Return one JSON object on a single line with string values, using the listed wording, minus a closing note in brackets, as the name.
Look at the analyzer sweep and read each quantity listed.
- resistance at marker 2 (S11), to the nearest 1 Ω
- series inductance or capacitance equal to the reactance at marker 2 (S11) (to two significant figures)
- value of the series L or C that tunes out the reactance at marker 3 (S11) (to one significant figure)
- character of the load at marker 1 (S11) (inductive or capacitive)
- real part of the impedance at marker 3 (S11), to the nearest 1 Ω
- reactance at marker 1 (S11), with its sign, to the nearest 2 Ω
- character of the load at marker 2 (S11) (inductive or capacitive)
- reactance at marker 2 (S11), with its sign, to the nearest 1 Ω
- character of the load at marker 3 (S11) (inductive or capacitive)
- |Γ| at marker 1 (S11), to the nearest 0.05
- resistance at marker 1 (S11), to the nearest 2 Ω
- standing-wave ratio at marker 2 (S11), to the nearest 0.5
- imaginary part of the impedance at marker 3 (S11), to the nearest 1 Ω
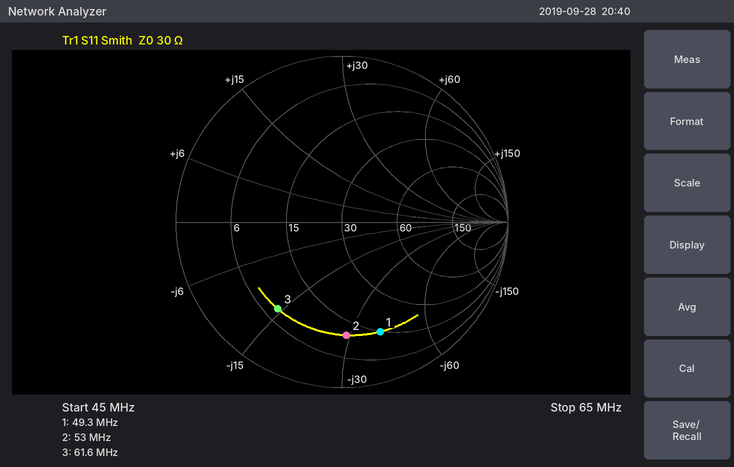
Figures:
{"resistance at marker 2 (S11), to the nearest 1 Ω": "11 Ω", "series inductance or capacitance equal to the reactance at marker 2 (S11)": "100 pF", "value of the series L or C that tunes out the reactance at marker 3 (S11)": "40 nH", "character of the load at marker 1 (S11)": "capacitive", "real part of the impedance at marker 3 (S11), to the nearest 1 Ω": "8 Ω", "reactance at marker 1 (S11), with its sign, to the nearest 2 Ω": "-38 Ω", "character of the load at marker 2 (S11)": "capacitive", "reactance at marker 2 (S11), with its sign, to the nearest 1 Ω": "-29 Ω", "character of the load at marker 3 (S11)": "capacitive", "|Γ| at marker 1 (S11), to the nearest 0.05": "0.70", "resistance at marker 1 (S11), to the nearest 2 Ω": "14 Ω", "standing-wave ratio at marker 2 (S11), to the nearest 0.5": "5.5", "imaginary part of the impedance at marker 3 (S11), to the nearest 1 Ω": "-14 Ω"}
